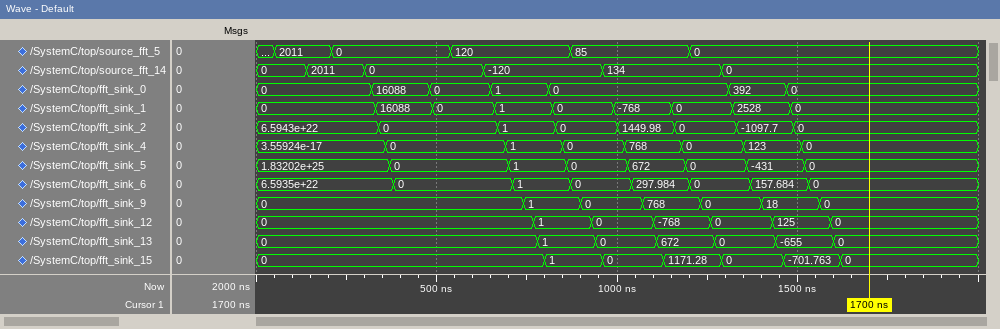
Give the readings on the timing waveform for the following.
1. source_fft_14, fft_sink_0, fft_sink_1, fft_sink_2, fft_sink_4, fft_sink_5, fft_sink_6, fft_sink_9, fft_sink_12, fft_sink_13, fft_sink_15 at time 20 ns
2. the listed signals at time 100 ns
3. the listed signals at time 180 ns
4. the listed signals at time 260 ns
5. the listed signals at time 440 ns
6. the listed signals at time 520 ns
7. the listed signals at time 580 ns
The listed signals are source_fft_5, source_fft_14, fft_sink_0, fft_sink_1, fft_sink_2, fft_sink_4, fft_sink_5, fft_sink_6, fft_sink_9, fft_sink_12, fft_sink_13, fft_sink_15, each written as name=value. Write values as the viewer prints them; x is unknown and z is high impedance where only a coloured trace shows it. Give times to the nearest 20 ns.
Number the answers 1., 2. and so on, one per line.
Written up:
1. source_fft_14=0, fft_sink_0=0, fft_sink_1=0, fft_sink_2=6.5943e+22, fft_sink_4=3.55924e-17, fft_sink_5=1.83202e+25, fft_sink_6=6.5935e+22, fft_sink_9=0, fft_sink_12=0, fft_sink_13=0, fft_sink_15=0
2. source_fft_5=2011, source_fft_14=0, fft_sink_0=0, fft_sink_1=0, fft_sink_2=6.5943e+22, fft_sink_4=3.55924e-17, fft_sink_5=1.83202e+25, fft_sink_6=6.5935e+22, fft_sink_9=0, fft_sink_12=0, fft_sink_13=0, fft_sink_15=0
3. source_fft_5=2011, source_fft_14=2011, fft_sink_0=0, fft_sink_1=0, fft_sink_2=6.5943e+22, fft_sink_4=3.55924e-17, fft_sink_5=1.83202e+25, fft_sink_6=6.5935e+22, fft_sink_9=0, fft_sink_12=0, fft_sink_13=0, fft_sink_15=0
4. source_fft_5=0, source_fft_14=2011, fft_sink_0=0, fft_sink_1=0, fft_sink_2=6.5943e+22, fft_sink_4=3.55924e-17, fft_sink_5=1.83202e+25, fft_sink_6=6.5935e+22, fft_sink_9=0, fft_sink_12=0, fft_sink_13=0, fft_sink_15=0
5. source_fft_5=0, source_fft_14=0, fft_sink_0=16088, fft_sink_1=16088, fft_sink_2=0, fft_sink_4=0, fft_sink_5=0, fft_sink_6=0, fft_sink_9=0, fft_sink_12=0, fft_sink_13=0, fft_sink_15=0
6. source_fft_5=0, source_fft_14=0, fft_sink_0=0, fft_sink_1=0, fft_sink_2=0, fft_sink_4=0, fft_sink_5=0, fft_sink_6=0, fft_sink_9=0, fft_sink_12=0, fft_sink_13=0, fft_sink_15=0
7. source_fft_5=120, source_fft_14=0, fft_sink_0=0, fft_sink_1=0, fft_sink_2=0, fft_sink_4=0, fft_sink_5=0, fft_sink_6=0, fft_sink_9=0, fft_sink_12=0, fft_sink_13=0, fft_sink_15=0
